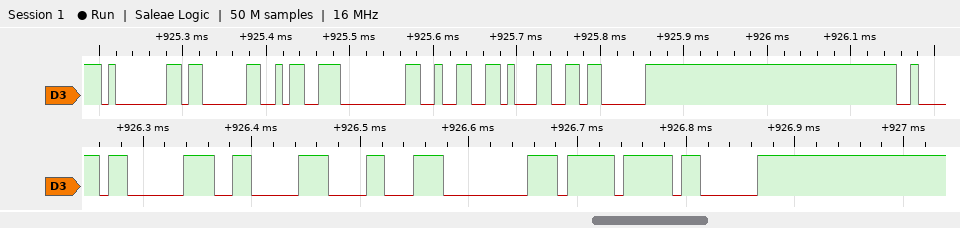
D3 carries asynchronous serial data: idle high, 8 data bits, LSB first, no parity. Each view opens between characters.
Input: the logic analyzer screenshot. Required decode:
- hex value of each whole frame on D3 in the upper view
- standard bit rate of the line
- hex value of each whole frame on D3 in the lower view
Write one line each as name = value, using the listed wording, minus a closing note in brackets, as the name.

hex value of each whole frame on D3 in the upper view = 01, 03, 9A, 00, 32, 31, 03
standard bit rate of the line = 115200 baud
hex value of each whole frame on D3 in the lower view = 03, 06, 18, 00, DF, 03
